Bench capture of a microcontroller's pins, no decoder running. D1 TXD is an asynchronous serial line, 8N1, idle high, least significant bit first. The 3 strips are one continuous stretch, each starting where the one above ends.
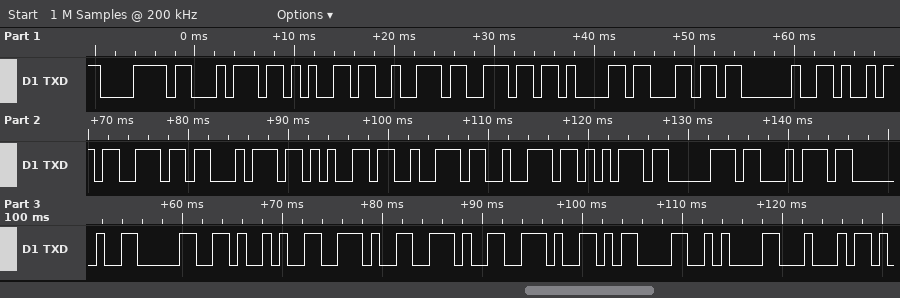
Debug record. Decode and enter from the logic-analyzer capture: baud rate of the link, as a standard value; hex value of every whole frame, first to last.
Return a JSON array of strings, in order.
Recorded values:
["1200 baud", "0x78 0x74 0x65 0x72 0x6E 0x61 0x6C 0x20 0x69 0x6E 0x74 0x65 0x72 0x72 0x75 0x70 0x74 0x20 0x30 0x29 0x2E 0x2E 0x2E 0x0D 0x0A 0x44"]
